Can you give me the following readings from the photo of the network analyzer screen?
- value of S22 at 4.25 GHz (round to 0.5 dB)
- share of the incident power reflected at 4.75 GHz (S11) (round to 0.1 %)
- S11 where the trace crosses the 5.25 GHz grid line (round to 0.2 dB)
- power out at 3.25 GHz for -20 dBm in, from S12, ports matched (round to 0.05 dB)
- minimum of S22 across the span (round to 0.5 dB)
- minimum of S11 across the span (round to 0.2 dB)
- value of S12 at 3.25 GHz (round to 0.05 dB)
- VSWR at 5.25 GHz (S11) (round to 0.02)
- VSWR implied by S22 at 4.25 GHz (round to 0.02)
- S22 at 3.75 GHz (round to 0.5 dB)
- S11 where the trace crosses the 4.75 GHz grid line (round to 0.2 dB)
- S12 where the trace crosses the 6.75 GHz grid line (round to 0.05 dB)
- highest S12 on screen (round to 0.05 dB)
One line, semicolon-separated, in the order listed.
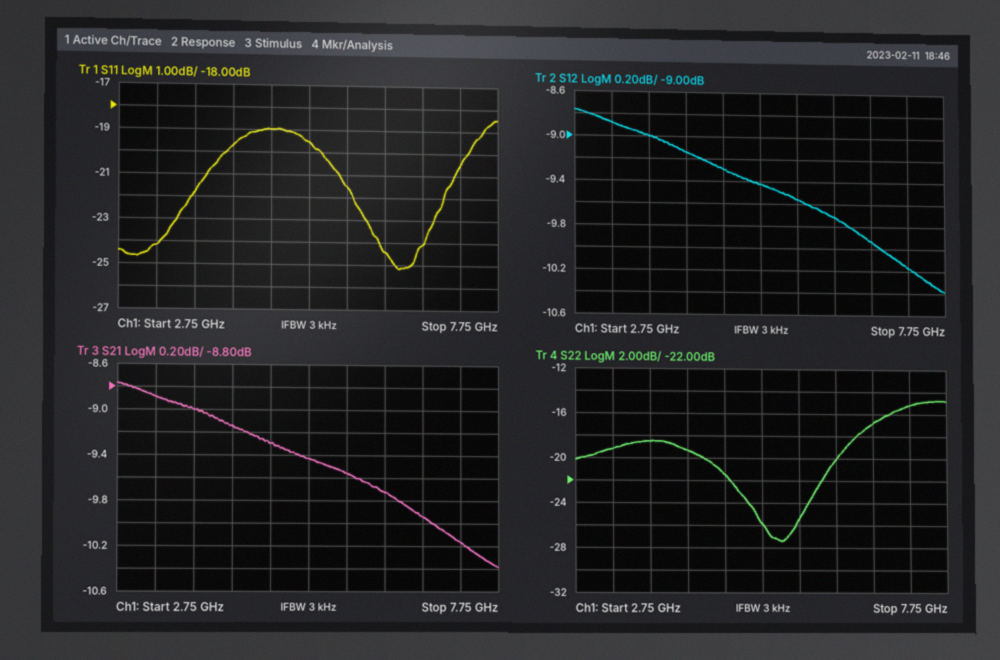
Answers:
-19.5 dB; 1.3 %; -19.6 dB; -28.90 dBm; -27.5 dB; -25.2 dB; -8.90 dB; 1.24; 1.24; -18.5 dB; -19.0 dB; -9.95 dB; -8.75 dB
